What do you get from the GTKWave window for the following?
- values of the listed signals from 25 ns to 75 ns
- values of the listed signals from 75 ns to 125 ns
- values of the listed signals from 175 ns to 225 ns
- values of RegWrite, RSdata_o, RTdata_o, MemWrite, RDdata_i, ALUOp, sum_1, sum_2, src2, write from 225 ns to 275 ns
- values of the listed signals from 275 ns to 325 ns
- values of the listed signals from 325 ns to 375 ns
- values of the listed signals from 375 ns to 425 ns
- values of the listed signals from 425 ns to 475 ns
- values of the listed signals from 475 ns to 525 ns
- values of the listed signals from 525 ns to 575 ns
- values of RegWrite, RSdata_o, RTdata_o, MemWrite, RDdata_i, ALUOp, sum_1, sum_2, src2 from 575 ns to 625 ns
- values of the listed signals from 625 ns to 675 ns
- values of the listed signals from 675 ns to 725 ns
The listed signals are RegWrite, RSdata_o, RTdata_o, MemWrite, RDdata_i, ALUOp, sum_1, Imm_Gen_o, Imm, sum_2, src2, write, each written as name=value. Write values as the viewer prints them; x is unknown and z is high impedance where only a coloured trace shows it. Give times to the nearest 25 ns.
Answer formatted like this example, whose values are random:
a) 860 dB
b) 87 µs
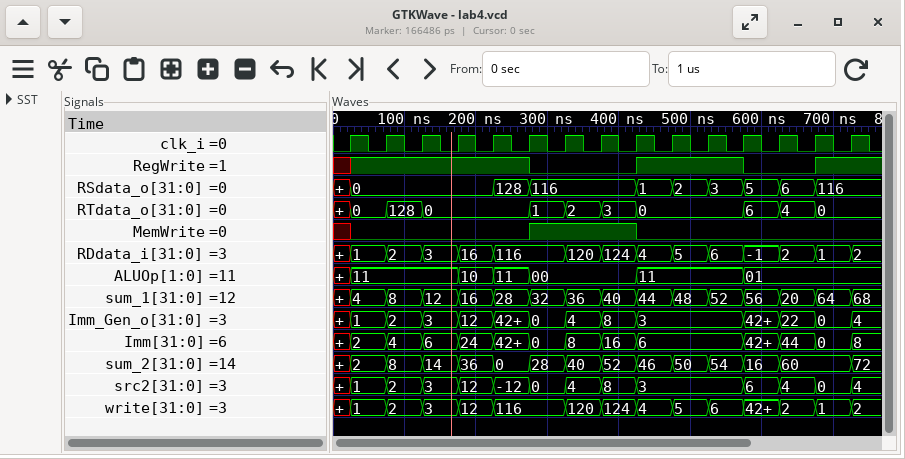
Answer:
a) RegWrite=1, RSdata_o=0, RTdata_o=0, MemWrite=0, RDdata_i=1, ALUOp=11, sum_1=4, Imm_Gen_o=1, Imm=2, sum_2=2, src2=1, write=1
b) RegWrite=1, RSdata_o=0, RTdata_o=128, MemWrite=0, RDdata_i=2, ALUOp=11, sum_1=8, Imm_Gen_o=2, Imm=4, sum_2=8, src2=2, write=2
c) RegWrite=1, RSdata_o=0, RTdata_o=0, MemWrite=0, RDdata_i=16, ALUOp=10, sum_1=16, Imm_Gen_o=12, Imm=24, sum_2=36, src2=12, write=12
d) RegWrite=1, RSdata_o=128, RTdata_o=0, MemWrite=0, RDdata_i=116, ALUOp=11, sum_1=28, sum_2=0, src2=-12, write=116
e) RegWrite=0, RSdata_o=116, RTdata_o=1, MemWrite=1, RDdata_i=116, ALUOp=00, sum_1=32, Imm_Gen_o=0, Imm=0, sum_2=28, src2=0, write=116
f) RegWrite=0, RSdata_o=116, RTdata_o=2, MemWrite=1, RDdata_i=120, ALUOp=00, sum_1=36, Imm_Gen_o=4, Imm=8, sum_2=40, src2=4, write=120
g) RegWrite=0, RSdata_o=116, RTdata_o=3, MemWrite=1, RDdata_i=124, ALUOp=00, sum_1=40, Imm_Gen_o=8, Imm=16, sum_2=52, src2=8, write=124
h) RegWrite=1, RSdata_o=1, RTdata_o=0, MemWrite=0, RDdata_i=4, ALUOp=11, sum_1=44, Imm_Gen_o=3, Imm=6, sum_2=46, src2=3, write=4
i) RegWrite=1, RSdata_o=2, RTdata_o=0, MemWrite=0, RDdata_i=5, ALUOp=11, sum_1=48, Imm_Gen_o=3, Imm=6, sum_2=50, src2=3, write=5
j) RegWrite=1, RSdata_o=3, RTdata_o=0, MemWrite=0, RDdata_i=6, ALUOp=11, sum_1=52, Imm_Gen_o=3, Imm=6, sum_2=54, src2=3, write=6
k) RegWrite=0, RSdata_o=5, RTdata_o=6, MemWrite=0, RDdata_i=-1, ALUOp=01, sum_1=56, sum_2=16, src2=6
l) RegWrite=0, RSdata_o=6, RTdata_o=4, MemWrite=0, RDdata_i=2, ALUOp=01, sum_1=20, Imm_Gen_o=22, Imm=44, sum_2=60, src2=4, write=2
m) RegWrite=1, RSdata_o=116, RTdata_o=0, MemWrite=0, RDdata_i=1, ALUOp=01, sum_1=64, Imm_Gen_o=0, Imm=0, sum_2=60, src2=0, write=1
